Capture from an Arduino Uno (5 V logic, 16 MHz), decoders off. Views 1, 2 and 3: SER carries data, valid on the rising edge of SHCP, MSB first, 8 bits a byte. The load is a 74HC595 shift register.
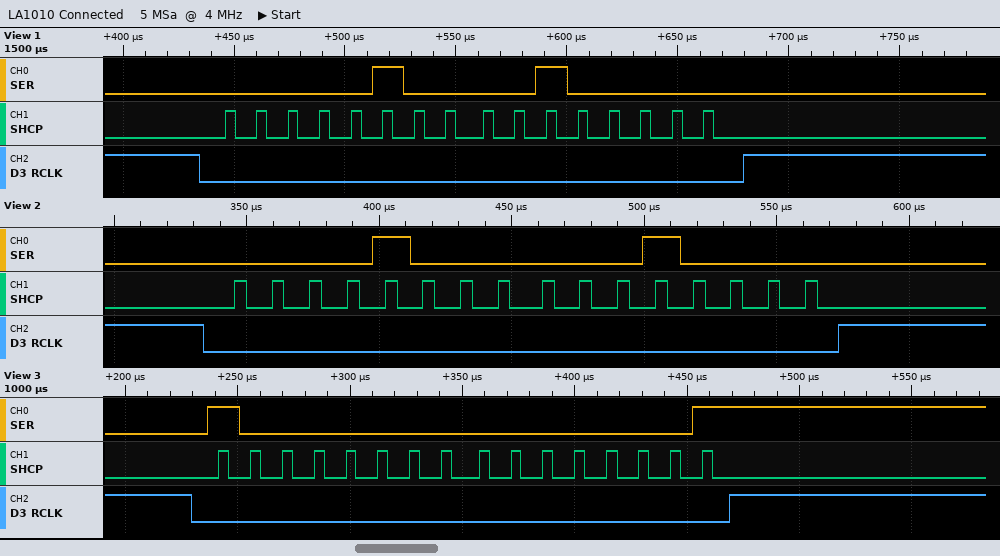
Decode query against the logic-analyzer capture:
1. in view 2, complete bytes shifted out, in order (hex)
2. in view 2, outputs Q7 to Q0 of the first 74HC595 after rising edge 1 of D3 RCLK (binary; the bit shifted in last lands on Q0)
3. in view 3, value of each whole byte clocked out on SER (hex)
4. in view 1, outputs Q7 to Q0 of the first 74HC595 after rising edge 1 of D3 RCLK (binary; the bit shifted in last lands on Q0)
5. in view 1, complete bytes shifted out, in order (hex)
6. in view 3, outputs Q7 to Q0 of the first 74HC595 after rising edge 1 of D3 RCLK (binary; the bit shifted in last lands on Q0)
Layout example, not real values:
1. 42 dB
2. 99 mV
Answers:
1. 08 10
2. 00010000
3. 0x80 0x01
4. 00100000
5. 04 20
6. 00000001
